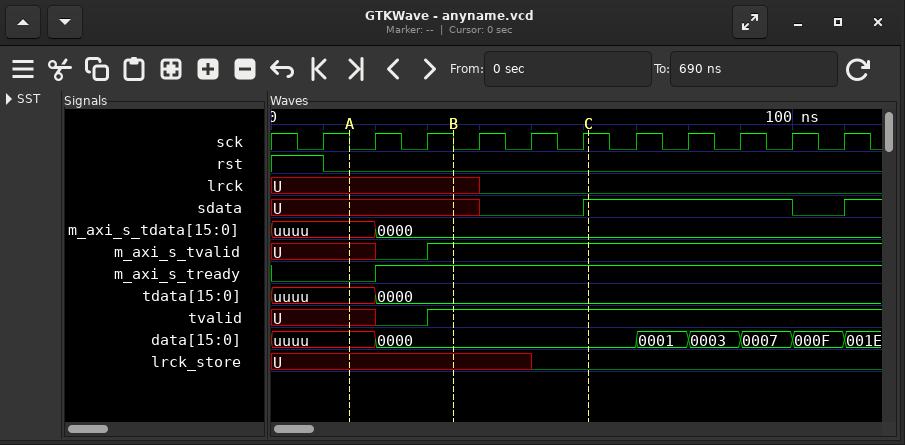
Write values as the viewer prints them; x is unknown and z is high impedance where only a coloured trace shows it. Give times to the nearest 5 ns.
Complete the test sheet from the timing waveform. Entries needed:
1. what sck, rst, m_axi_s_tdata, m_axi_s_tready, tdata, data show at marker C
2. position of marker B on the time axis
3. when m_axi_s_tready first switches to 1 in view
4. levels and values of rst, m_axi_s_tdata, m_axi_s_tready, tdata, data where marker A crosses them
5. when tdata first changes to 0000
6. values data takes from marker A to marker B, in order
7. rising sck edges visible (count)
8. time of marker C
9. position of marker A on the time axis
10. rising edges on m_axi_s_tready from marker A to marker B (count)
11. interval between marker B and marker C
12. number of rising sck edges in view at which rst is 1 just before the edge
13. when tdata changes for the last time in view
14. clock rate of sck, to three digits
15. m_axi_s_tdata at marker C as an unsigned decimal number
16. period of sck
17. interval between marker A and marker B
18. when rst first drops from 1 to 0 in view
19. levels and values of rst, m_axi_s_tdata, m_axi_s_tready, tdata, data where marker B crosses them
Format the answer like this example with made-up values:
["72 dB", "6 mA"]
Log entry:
["sck=1, rst=0, m_axi_s_tdata=0000, m_axi_s_tready=1, tdata=0000, data=0000", "35 ns", "20 ns", "rst=0, m_axi_s_tdata=uuuu, m_axi_s_tready=0, tdata=uuuu, data=uuuu", "20 ns", "uuuu, 0000", "11", "60 ns", "15 ns", "1", "25 ns", "1", "20 ns", "100 MHz", "0", "10 ns", "20 ns", "10 ns", "rst=0, m_axi_s_tdata=0000, m_axi_s_tready=1, tdata=0000, data=0000"]
